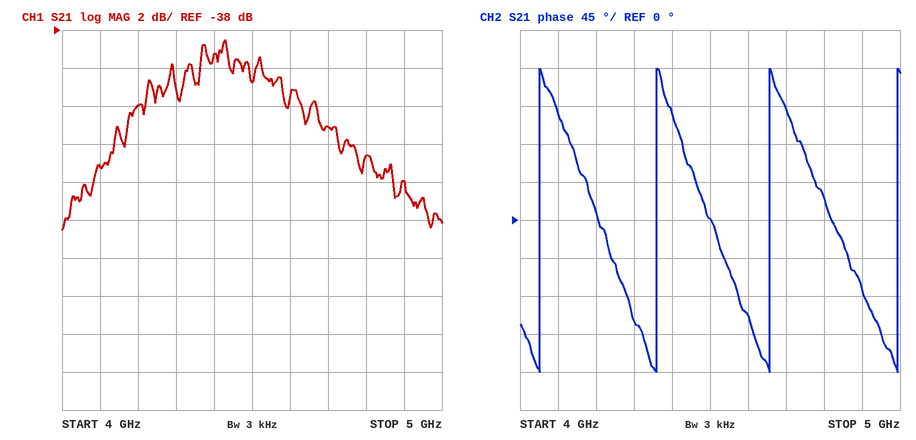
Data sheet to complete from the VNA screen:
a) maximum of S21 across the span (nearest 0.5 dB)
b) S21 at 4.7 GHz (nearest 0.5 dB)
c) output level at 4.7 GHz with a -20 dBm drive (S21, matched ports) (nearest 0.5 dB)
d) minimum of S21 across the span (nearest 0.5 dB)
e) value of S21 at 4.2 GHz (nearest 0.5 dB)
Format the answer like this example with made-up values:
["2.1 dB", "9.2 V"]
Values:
["-38.5 dB", "-43.0 dB", "-63.0 dBm", "-48.5 dB", "-42.0 dB"]
